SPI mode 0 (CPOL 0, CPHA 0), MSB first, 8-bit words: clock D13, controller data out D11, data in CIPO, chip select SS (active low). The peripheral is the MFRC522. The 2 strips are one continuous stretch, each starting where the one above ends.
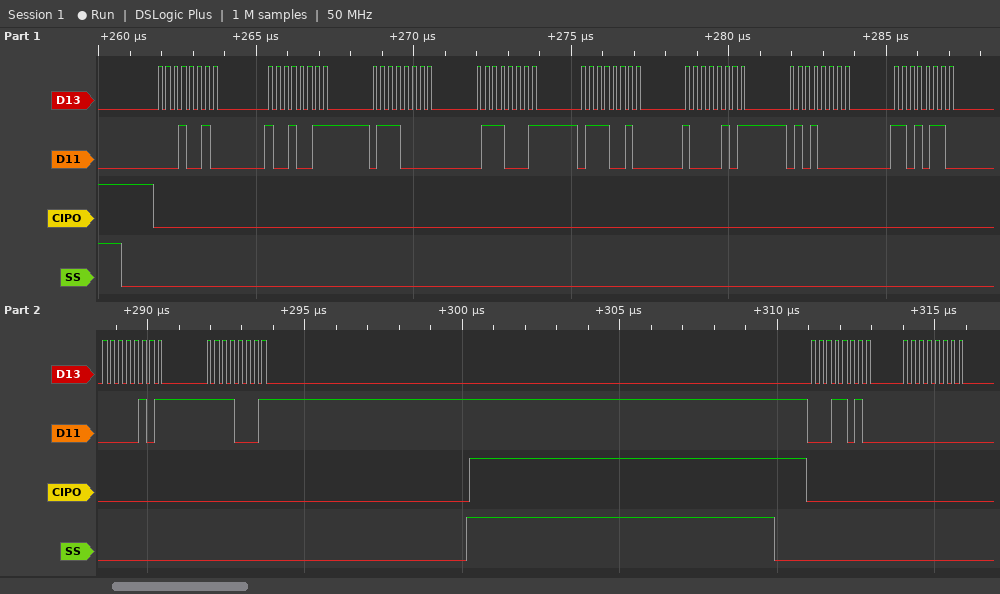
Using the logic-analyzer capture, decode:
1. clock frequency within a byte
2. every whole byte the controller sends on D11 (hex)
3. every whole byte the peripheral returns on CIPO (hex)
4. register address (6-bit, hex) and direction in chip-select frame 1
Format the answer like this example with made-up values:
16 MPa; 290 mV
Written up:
4 MHz; 12 93 70 71 72 85 50 D6 05 F1 1A 00; 00 00 00 00 00 00 00 00 00 00 00 00; 0x09 write
